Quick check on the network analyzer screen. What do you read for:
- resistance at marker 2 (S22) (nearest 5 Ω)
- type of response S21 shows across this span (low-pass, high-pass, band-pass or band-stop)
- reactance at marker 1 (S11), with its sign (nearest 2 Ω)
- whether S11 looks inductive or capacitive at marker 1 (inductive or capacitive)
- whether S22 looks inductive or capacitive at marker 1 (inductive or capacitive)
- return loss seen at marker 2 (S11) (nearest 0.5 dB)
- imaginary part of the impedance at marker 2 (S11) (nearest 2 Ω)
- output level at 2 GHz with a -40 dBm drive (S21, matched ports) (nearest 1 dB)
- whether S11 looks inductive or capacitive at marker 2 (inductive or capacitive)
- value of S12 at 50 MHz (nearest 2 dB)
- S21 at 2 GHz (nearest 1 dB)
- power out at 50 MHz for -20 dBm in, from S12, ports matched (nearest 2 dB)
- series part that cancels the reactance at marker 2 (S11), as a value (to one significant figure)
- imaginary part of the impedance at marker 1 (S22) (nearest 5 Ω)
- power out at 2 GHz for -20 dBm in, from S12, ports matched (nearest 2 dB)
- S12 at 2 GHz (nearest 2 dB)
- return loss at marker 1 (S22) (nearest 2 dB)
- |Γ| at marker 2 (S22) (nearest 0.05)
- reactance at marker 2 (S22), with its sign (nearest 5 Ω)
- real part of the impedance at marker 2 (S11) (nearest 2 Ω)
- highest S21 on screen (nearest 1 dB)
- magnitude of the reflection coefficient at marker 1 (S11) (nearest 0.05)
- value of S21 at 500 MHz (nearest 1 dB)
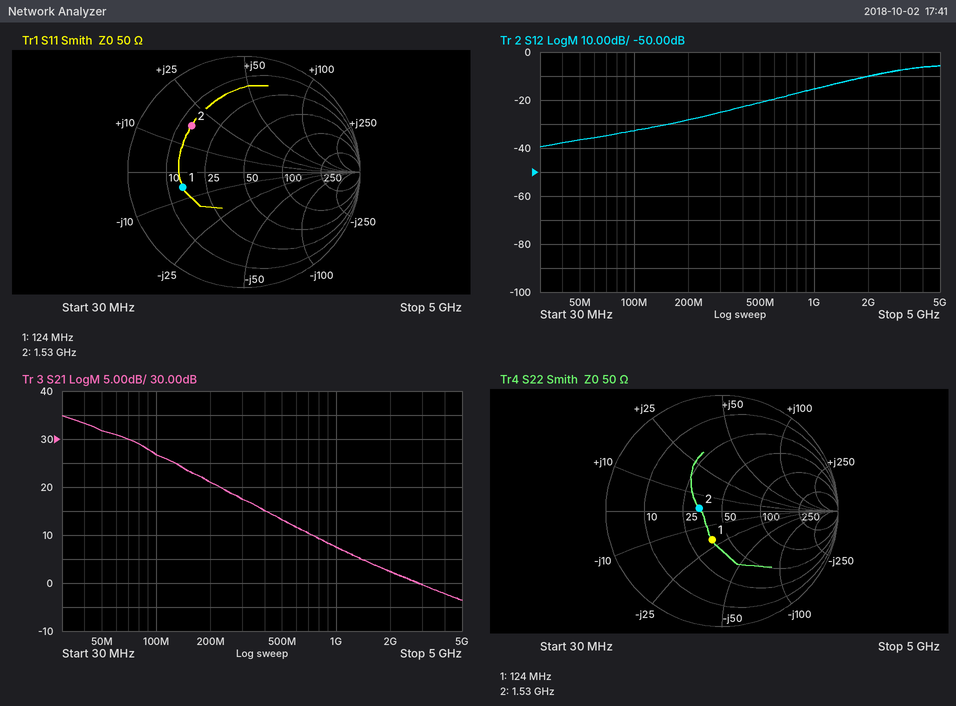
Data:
35 Ω
low-pass
-6 Ω
capacitive
capacitive
4.5 dB
+18 Ω
-38 dBm
inductive
-36 dB
2 dB
-56 dBm
6 pF
-20 Ω
-30 dBm
-10 dB
12 dB
0.20
0 Ω
14 Ω
35 dB
0.55
13 dB
